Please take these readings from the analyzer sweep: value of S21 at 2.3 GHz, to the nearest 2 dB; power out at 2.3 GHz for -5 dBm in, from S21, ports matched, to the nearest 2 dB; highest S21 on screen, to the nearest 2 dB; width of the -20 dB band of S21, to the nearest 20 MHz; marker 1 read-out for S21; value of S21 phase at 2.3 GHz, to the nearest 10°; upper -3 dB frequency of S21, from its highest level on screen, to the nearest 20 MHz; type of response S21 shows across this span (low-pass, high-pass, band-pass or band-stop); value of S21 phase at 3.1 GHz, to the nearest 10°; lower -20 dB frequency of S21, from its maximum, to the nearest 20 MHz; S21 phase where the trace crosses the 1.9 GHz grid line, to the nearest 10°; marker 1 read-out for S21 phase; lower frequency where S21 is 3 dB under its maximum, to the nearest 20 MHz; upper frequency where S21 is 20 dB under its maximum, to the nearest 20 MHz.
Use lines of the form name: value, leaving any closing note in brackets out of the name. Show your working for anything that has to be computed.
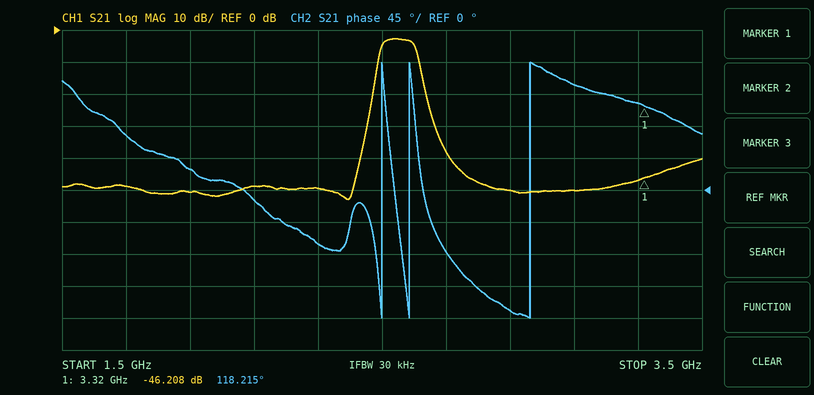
value of S21 at 2.3 GHz, to the nearest 2 dB: -50 dB
power out at 2.3 GHz for -5 dBm in, from S21, ports matched, to the nearest 2 dB: -5 dBm + (-50 dB) = -54 dBm
highest S21 on screen, to the nearest 2 dB: -2 dB
width of the -20 dB band of S21, to the nearest 20 MHz: 2.64 GHz − 2.46 GHz = 180 MHz
marker 1 read-out for S21: -46.208 dB
value of S21 phase at 2.3 GHz, to the nearest 10°: -80°
upper -3 dB frequency of S21, from its highest level on screen, to the nearest 20 MHz: 2.60 GHz
type of response S21 shows across this span: band-pass
value of S21 phase at 3.1 GHz, to the nearest 10°: 150°
lower -20 dB frequency of S21, from its maximum, to the nearest 20 MHz: 2.46 GHz
S21 phase where the trace crosses the 1.9 GHz grid line, to the nearest 10°: 30°
marker 1 read-out for S21 phase: 118.215°
lower frequency where S21 is 3 dB under its maximum, to the nearest 20 MHz: 2.50 GHz
upper frequency where S21 is 20 dB under its maximum, to the nearest 20 MHz: 2.64 GHz
